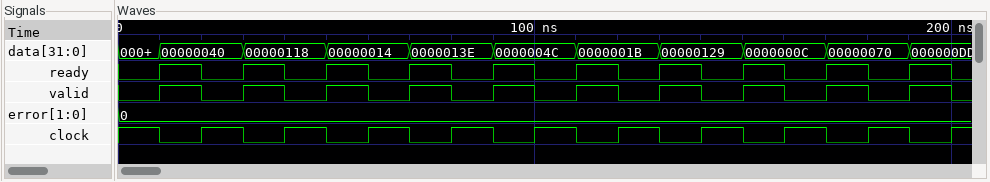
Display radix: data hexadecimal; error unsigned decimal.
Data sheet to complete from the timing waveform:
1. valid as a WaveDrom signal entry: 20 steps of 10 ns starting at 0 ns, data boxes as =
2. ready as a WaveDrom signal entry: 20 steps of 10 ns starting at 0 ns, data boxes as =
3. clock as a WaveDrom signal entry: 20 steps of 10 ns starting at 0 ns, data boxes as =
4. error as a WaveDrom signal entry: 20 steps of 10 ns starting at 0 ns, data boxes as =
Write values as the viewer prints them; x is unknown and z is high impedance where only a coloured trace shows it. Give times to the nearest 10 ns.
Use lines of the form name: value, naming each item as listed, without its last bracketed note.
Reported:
valid as a WaveDrom signal entry: 20 steps of 10 ns starting at 0 ns, data boxes as =: {name: 'valid', wave: '01010101010101010101'}
ready as a WaveDrom signal entry: 20 steps of 10 ns starting at 0 ns, data boxes as =: {name: 'ready', wave: '01010101010101010101'}
clock as a WaveDrom signal entry: 20 steps of 10 ns starting at 0 ns, data boxes as =: {name: 'clock', wave: '10101010101010101010'}
error as a WaveDrom signal entry: 20 steps of 10 ns starting at 0 ns, data boxes as =: {name: 'error', wave: '=...................', data: '0'}
